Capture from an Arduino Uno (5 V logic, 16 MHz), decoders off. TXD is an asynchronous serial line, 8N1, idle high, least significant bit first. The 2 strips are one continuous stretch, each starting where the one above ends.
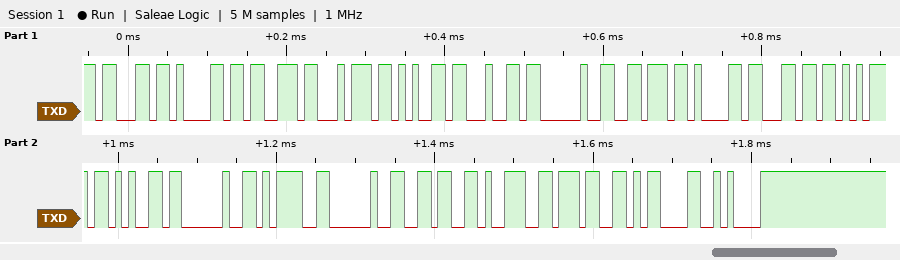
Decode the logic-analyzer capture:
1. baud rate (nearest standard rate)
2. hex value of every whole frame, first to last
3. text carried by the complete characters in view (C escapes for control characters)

115200 baud
63 61 73 74 65 64 20 76 61 6C 75 65 20 3D 20 36 39 37 0D 0A
"casted value = 697\r\n"
